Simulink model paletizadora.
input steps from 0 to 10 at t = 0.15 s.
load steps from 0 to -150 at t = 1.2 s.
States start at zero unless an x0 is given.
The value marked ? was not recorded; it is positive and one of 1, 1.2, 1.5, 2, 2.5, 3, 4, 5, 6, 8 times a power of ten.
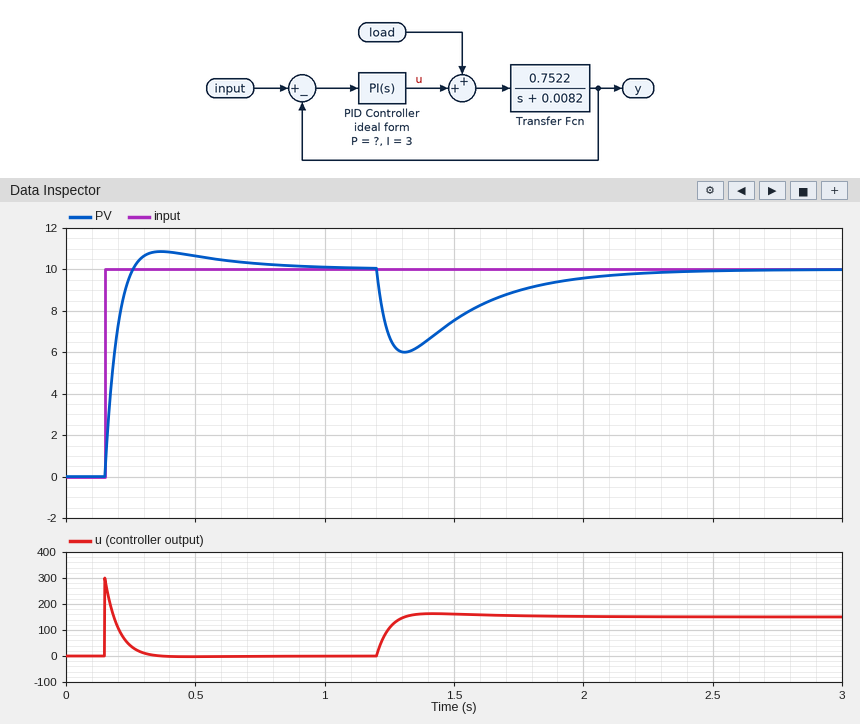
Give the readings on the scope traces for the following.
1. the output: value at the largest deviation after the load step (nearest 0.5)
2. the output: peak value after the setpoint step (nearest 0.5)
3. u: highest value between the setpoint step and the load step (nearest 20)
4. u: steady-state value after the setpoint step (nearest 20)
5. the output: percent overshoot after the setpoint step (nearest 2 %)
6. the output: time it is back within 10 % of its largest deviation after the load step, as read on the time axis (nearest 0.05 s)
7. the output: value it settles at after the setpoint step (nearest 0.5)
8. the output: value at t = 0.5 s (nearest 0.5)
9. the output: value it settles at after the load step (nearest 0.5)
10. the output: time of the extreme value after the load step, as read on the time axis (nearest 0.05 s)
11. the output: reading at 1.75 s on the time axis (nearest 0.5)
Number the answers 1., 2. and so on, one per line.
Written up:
1. 6.0
2. 11.0
3. 300
4. 0
5. 8 %
6. 2.00 s
7. 10.0
8. 10.5
9. 10.0
10. 1.30 s
11. 9.0
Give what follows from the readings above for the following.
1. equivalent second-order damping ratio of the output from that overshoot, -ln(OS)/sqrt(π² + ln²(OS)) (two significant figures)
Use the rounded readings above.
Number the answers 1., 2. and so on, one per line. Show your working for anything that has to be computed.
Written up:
1. ln(0.08) = -2.526; 2.526 / sqrt(9.870 + 6.379) = 0.63
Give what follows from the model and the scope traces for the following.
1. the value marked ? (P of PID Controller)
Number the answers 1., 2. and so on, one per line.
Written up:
1. 30
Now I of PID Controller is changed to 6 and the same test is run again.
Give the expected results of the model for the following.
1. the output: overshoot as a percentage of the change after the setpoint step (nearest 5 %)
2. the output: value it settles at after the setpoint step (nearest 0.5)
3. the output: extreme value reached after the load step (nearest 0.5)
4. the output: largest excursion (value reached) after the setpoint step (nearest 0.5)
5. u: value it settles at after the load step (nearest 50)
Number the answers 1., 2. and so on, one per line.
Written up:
1. 15 %
2. 10.0
3. 6.5
4. 11.5
5. 150
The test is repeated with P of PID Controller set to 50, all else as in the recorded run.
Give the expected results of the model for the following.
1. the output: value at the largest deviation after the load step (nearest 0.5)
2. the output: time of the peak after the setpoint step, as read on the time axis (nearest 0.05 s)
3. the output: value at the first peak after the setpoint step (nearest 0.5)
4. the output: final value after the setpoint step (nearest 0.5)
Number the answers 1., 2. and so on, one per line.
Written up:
1. 7.5
2. 0.30 s
3. 10.5
4. 10.0
